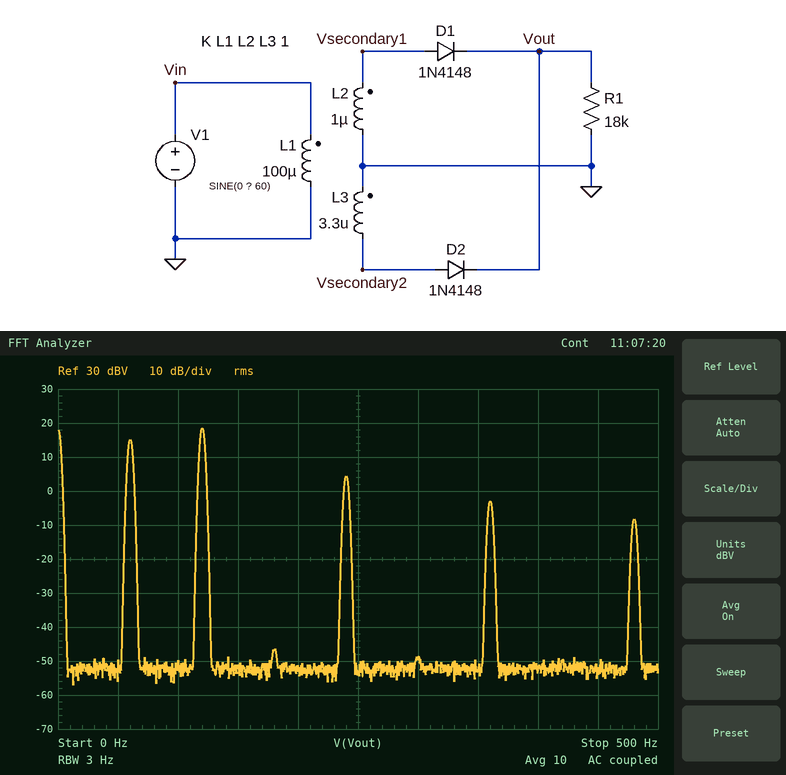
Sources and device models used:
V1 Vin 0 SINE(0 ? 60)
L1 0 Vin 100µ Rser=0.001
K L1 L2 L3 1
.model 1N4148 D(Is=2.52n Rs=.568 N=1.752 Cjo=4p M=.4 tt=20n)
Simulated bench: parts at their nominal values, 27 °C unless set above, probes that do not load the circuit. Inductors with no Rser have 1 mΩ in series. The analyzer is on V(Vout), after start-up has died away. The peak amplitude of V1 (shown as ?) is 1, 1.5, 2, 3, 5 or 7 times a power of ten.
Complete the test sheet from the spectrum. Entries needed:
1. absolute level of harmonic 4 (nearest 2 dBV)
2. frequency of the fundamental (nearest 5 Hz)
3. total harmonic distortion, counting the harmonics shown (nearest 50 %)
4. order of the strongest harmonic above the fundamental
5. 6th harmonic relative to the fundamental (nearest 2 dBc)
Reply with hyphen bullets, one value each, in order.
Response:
- 4 dBV
- 60 Hz
- 150 %
- 2
- -18 dBc
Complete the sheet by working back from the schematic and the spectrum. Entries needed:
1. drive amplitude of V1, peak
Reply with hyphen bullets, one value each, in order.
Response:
- 200 V
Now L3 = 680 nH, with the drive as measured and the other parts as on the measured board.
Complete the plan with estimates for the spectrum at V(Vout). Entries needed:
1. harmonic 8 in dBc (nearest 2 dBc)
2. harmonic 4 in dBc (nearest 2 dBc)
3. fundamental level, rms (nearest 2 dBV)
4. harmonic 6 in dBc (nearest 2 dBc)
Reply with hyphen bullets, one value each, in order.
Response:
- -14 dBc
- -2 dBc
- 2 dBV
- -8 dBc
